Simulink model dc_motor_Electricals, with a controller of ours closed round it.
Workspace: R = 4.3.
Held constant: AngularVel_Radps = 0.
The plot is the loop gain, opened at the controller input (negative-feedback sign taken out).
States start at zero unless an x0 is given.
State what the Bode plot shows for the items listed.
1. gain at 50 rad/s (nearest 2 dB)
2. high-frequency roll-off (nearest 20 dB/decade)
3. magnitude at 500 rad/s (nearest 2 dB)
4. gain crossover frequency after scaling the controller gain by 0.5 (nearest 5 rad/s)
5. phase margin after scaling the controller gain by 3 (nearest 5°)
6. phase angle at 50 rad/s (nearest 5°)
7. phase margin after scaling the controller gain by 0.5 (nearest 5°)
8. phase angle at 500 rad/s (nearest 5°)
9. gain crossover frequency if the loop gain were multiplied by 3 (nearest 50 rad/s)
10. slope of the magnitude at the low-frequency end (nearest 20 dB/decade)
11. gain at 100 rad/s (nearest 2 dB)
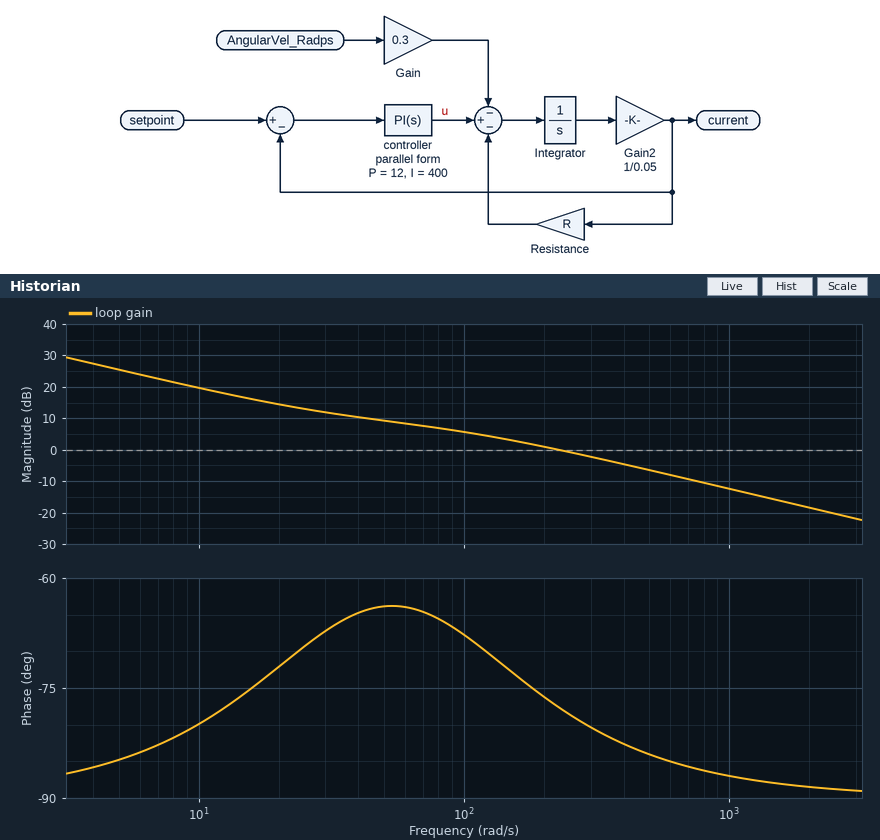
10 dB
-20 dB/decade
-6 dB
95 rad/s
95°
-65°
115°
-85°
700 rad/s
-20 dB/decade
6 dB
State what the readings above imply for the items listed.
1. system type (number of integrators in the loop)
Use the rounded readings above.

1
